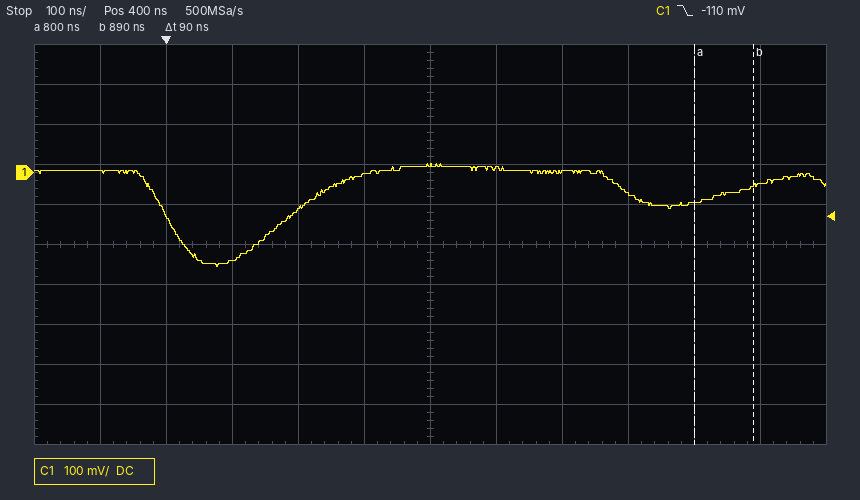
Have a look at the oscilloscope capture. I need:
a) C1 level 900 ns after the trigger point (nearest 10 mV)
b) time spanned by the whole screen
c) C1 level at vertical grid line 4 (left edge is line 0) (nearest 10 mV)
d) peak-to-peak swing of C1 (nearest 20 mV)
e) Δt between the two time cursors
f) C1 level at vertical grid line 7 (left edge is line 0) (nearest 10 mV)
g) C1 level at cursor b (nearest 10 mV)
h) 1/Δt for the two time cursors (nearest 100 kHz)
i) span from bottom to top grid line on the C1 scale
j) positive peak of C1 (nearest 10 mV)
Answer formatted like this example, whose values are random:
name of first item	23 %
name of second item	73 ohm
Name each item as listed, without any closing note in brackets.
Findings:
C1 level 900 ns after the trigger point	-30 mV
time spanned by the whole screen	1.2 µs
C1 level at vertical grid line 4 (left edge is line 0)	-90 mV
peak-to-peak swing of C1	260 mV
Δt between the two time cursors	90 ns
C1 level at vertical grid line 7 (left edge is line 0)	10 mV
C1 level at cursor b	-30 mV
1/Δt for the two time cursors	11.1 MHz
span from bottom to top grid line on the C1 scale	1 V
positive peak of C1	20 mV
